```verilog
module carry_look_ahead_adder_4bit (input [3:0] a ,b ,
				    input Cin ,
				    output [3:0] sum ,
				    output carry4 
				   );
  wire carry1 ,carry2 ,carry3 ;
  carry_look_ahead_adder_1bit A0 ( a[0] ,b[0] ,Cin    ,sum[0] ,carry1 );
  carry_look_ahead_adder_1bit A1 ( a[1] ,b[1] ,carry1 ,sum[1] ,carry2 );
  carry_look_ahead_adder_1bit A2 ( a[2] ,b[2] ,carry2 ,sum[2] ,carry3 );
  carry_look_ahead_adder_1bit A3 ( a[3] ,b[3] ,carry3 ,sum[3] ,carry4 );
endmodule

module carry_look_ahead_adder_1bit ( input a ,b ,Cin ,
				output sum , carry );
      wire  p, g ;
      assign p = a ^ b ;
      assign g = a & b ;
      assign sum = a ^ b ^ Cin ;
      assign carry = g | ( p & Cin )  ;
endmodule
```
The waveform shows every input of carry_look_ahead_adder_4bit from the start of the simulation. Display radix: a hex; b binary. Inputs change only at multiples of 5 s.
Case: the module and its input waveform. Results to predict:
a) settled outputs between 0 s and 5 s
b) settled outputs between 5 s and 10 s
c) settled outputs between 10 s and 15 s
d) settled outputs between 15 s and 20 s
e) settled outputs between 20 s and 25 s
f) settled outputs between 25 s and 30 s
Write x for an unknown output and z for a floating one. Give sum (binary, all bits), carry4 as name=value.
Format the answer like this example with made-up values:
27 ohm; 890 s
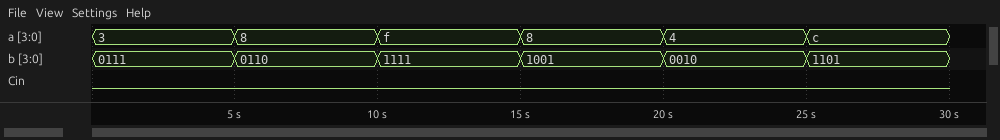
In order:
sum=1010, carry4=0; sum=1110, carry4=0; sum=1110, carry4=1; sum=0001, carry4=1; sum=0110, carry4=0; sum=1001, carry4=1
